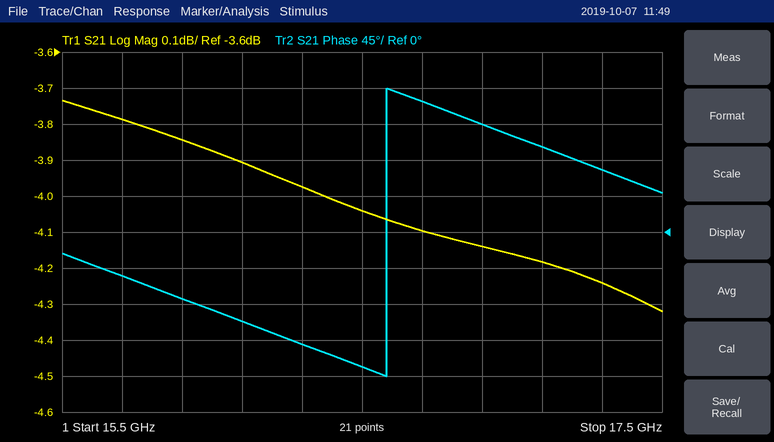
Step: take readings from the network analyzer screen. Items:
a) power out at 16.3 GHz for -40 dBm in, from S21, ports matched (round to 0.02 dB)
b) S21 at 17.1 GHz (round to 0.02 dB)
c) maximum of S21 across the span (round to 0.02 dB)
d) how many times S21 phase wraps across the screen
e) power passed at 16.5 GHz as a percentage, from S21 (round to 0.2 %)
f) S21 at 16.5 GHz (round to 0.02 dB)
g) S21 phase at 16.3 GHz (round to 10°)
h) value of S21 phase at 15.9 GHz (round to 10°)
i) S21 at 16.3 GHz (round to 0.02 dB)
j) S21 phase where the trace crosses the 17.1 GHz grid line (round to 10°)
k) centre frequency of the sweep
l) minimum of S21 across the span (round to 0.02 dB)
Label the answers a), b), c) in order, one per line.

a) -43.98 dBm
b) -4.18 dB
c) -3.74 dB
d) 1
e) 39.4 %
f) -4.04 dB
g) -140°
h) -80°
i) -3.98 dB
j) 110°
k) 16.5 GHz
l) -4.32 dB
